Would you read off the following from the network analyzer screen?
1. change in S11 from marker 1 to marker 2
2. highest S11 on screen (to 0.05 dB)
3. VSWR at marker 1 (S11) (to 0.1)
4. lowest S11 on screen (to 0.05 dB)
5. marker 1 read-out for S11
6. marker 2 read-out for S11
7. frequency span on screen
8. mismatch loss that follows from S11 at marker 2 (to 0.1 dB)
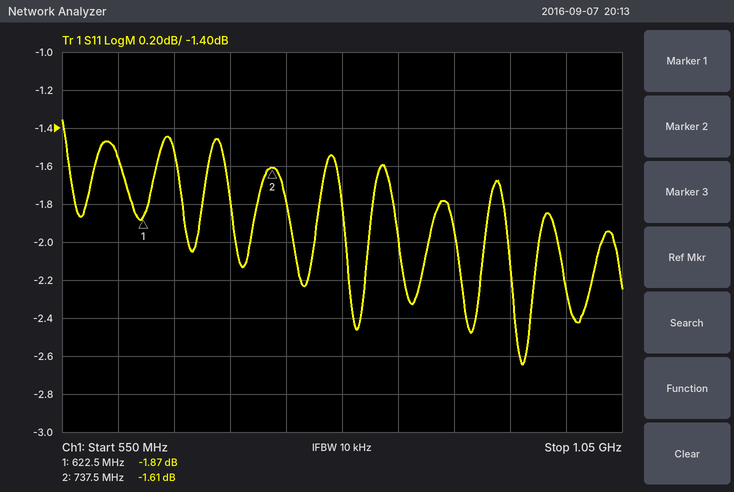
0.26 dB
-1.35 dB
9.3
-2.65 dB
-1.87 dB
-1.61 dB
500 MHz
5.1 dB
